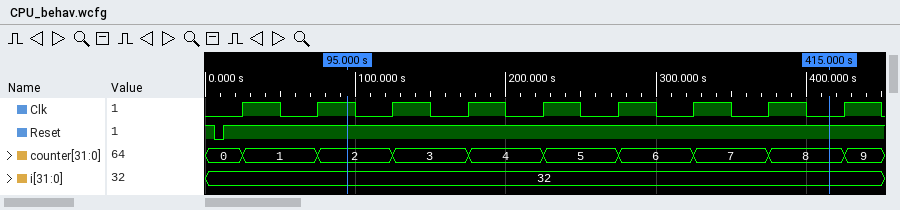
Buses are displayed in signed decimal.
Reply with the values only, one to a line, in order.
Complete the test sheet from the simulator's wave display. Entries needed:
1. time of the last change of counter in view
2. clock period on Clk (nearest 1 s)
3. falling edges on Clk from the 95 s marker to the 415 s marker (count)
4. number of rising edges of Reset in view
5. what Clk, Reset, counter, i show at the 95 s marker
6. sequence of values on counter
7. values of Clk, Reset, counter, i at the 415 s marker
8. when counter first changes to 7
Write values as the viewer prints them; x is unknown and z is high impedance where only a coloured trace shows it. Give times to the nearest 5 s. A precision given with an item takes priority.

425 s
50 s
7
1
Clk=1, Reset=1, counter=2, i=32
0, 1, 2, 3, 4, 5, 6, 7, 8, 9
Clk=0, Reset=1, counter=8, i=32
325 s
